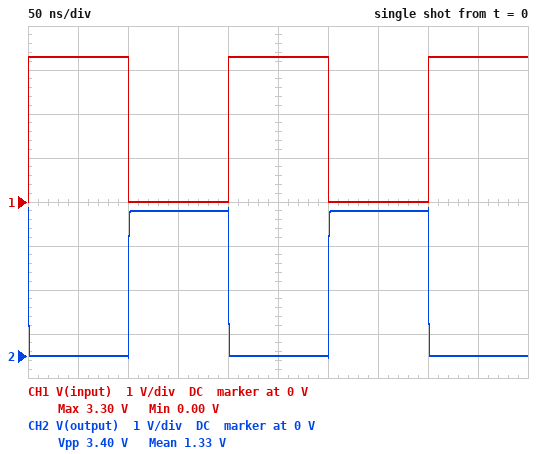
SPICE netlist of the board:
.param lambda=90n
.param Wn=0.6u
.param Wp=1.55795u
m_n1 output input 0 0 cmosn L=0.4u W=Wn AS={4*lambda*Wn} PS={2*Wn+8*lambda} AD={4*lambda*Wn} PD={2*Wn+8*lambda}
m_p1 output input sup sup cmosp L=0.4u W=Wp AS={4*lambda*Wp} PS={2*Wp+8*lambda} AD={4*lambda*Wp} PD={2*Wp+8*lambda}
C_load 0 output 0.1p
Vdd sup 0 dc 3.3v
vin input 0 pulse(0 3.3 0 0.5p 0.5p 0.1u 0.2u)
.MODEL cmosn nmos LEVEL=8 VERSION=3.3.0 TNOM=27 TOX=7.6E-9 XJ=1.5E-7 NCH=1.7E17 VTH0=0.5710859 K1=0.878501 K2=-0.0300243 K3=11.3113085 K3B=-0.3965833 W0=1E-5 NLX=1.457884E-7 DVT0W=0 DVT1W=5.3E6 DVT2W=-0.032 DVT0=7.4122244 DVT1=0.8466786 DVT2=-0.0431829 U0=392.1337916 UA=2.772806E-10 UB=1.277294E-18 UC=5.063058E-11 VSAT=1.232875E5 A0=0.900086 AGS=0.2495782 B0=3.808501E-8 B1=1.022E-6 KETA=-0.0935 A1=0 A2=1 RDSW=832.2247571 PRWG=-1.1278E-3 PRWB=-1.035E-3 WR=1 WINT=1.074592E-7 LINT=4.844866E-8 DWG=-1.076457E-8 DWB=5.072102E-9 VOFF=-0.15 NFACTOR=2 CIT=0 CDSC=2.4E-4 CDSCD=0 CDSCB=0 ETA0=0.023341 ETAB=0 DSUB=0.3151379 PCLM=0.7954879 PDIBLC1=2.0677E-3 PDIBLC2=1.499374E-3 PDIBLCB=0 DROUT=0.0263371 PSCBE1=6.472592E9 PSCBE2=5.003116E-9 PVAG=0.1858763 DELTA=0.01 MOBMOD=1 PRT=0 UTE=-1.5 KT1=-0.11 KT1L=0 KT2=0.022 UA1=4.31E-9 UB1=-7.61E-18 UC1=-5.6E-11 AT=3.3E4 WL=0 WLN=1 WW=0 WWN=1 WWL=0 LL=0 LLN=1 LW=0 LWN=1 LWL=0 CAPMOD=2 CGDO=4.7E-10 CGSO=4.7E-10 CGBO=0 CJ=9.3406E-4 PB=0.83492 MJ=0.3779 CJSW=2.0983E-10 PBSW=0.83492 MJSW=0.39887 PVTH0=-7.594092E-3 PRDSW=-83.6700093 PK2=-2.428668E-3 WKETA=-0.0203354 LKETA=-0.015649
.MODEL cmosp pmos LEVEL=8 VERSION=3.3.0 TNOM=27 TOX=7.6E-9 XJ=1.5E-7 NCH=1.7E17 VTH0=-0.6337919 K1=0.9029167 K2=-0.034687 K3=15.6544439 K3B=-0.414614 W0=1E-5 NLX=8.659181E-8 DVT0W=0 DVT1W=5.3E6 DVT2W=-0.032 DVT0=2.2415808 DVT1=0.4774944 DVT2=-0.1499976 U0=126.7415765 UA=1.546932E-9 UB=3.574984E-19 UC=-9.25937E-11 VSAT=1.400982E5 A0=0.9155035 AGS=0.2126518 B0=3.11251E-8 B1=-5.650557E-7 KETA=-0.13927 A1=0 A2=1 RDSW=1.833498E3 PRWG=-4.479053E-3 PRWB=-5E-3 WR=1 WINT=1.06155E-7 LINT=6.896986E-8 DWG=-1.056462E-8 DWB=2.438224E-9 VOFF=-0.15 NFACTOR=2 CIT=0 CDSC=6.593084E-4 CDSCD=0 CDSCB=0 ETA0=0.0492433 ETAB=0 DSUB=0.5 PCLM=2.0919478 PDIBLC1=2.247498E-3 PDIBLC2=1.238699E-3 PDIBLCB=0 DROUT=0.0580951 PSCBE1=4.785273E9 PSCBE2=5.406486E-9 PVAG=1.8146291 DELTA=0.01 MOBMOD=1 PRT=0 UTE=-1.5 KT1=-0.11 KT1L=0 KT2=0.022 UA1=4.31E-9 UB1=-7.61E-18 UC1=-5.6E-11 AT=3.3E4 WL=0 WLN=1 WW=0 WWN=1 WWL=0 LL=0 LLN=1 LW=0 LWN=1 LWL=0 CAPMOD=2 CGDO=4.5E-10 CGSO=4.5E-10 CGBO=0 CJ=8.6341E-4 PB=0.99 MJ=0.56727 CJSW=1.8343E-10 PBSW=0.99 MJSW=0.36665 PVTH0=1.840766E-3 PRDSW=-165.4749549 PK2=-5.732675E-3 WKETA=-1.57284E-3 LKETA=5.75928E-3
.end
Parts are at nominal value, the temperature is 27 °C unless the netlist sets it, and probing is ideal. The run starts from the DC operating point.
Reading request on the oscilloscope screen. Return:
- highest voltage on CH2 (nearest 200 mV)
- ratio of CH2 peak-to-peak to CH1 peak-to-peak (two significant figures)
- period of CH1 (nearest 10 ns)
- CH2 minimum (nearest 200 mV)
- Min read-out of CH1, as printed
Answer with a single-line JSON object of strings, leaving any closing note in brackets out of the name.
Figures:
{"highest voltage on CH2": "3.4 V", "ratio of CH2 peak-to-peak to CH1 peak-to-peak": "1.0", "period of CH1": "200 ns", "CH2 minimum": "0 V", "Min read-out of CH1, as printed": "0.00 V"}
